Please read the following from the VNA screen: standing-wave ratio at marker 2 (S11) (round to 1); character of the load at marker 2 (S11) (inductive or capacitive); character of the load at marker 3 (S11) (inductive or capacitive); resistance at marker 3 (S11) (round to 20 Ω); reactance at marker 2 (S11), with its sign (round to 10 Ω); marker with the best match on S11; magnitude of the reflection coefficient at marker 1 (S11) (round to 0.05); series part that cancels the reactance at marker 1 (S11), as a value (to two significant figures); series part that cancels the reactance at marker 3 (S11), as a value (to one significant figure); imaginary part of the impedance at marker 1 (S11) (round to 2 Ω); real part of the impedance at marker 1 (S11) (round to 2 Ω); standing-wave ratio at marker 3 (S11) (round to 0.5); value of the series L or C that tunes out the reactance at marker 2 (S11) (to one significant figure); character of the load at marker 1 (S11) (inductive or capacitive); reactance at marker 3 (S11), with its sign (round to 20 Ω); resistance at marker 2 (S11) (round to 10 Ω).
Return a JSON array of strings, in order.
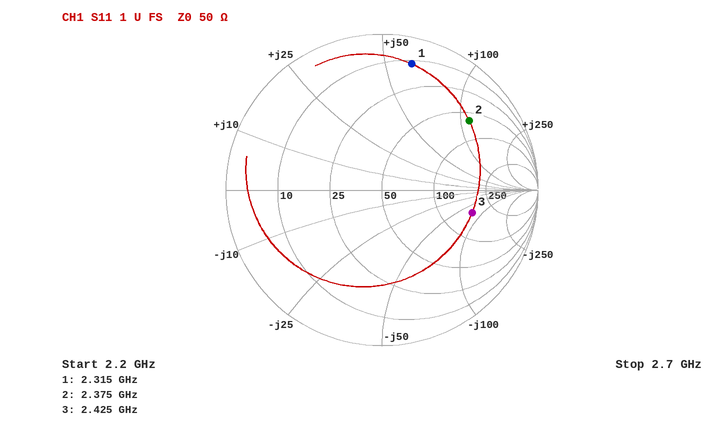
["6", "inductive", "capacitive", "160 Ω", "+110 Ω", "marker 3", "0.85", "1.1 pF", "5 nH", "+62 Ω", "12 Ω", "4.0", "600 fF", "inductive", "-80 Ω", "60 Ω"]
